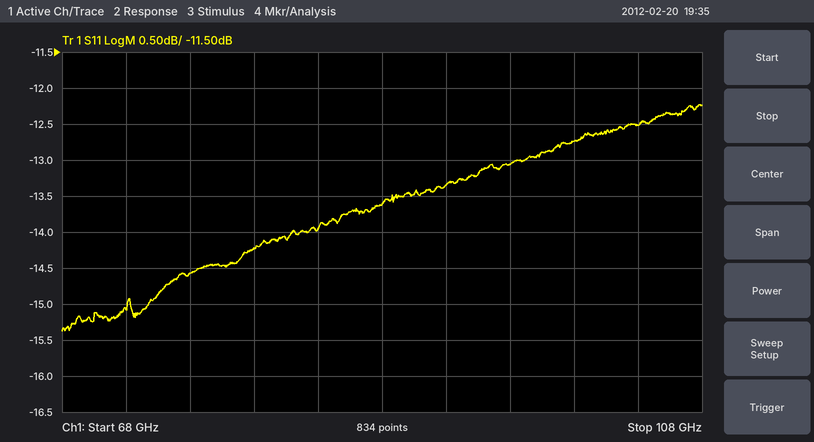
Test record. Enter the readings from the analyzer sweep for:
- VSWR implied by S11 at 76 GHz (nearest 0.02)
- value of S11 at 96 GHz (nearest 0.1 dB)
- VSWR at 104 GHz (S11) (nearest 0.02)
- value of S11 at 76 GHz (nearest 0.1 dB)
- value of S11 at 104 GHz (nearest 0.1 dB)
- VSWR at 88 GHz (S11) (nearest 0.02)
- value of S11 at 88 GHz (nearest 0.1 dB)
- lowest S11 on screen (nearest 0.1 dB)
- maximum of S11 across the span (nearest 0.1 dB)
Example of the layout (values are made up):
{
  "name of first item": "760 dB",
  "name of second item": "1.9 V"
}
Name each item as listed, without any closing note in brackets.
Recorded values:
{
  "VSWR implied by S11 at 76 GHz": "1.46",
  "value of S11 at 96 GHz": "-13.1 dB",
  "VSWR at 104 GHz (S11)": "1.62",
  "value of S11 at 76 GHz": "-14.6 dB",
  "value of S11 at 104 GHz": "-12.5 dB",
  "VSWR at 88 GHz (S11)": "1.52",
  "value of S11 at 88 GHz": "-13.6 dB",
  "lowest S11 on screen": "-15.4 dB",
  "maximum of S11 across the span": "-12.2 dB"
}
